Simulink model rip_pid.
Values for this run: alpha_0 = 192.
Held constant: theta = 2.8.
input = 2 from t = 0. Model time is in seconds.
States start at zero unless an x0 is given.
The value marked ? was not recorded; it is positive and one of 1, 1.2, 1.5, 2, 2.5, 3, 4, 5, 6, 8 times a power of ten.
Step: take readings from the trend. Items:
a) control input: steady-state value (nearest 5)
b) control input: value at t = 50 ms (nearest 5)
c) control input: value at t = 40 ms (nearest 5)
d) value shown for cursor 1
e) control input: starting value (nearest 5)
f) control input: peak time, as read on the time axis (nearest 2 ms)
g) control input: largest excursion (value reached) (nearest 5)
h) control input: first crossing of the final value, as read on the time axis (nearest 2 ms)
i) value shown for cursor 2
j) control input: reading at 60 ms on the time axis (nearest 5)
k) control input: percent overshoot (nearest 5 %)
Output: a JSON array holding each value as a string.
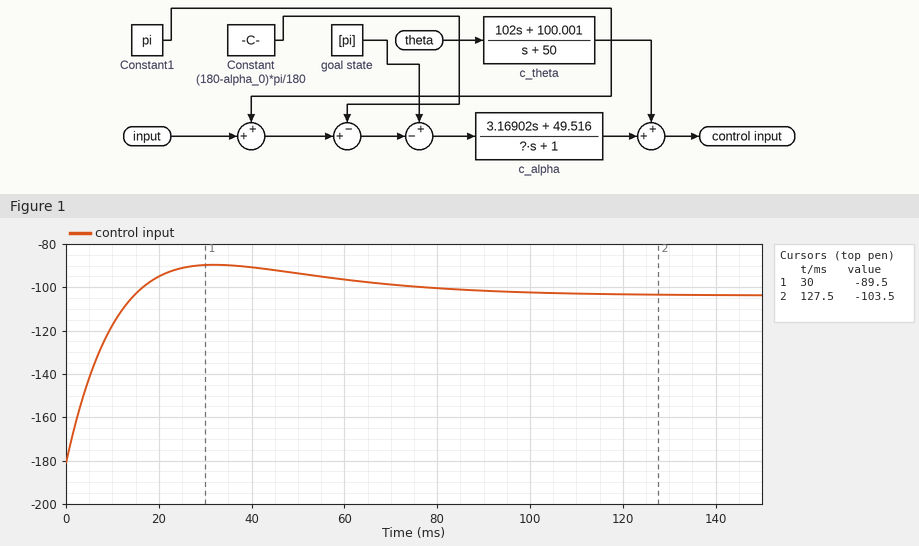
["-105", "-95", "-90", "-89.5", "-180", "32 ms", "-90", "14 ms", "-103.5", "-95", "20 %"]
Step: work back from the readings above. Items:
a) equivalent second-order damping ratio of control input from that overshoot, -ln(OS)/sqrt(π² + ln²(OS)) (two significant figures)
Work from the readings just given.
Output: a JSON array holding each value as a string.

["0.46"]
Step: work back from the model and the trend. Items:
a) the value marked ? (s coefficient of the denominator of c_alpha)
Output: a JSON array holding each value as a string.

["0.015"]
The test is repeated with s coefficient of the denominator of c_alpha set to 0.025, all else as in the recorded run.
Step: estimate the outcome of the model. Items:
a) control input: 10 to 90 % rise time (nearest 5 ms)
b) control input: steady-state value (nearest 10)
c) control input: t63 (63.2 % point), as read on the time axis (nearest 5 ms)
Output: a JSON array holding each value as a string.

["30 ms", "-100", "15 ms"]
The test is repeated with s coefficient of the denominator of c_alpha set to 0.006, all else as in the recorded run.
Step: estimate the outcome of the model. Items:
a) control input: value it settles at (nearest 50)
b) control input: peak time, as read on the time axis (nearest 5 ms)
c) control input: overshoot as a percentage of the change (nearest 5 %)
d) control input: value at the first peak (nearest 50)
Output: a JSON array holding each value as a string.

["-100", "20 ms", "10 %", "-50"]
